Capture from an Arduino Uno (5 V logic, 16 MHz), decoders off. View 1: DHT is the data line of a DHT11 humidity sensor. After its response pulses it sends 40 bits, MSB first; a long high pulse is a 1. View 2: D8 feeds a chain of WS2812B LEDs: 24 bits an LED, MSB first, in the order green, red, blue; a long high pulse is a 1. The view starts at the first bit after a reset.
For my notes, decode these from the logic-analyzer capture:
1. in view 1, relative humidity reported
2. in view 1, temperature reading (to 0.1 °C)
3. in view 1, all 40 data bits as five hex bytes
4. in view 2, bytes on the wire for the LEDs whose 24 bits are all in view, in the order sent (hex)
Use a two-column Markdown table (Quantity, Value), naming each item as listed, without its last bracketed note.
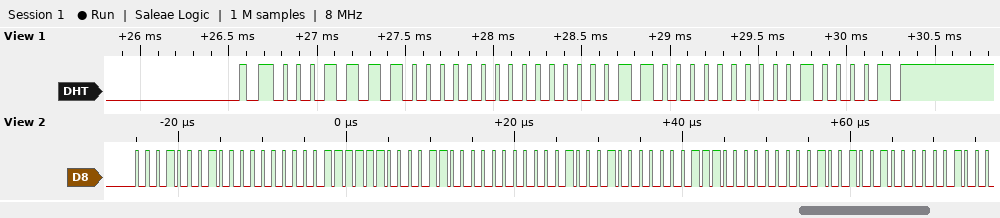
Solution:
| Quantity | Value |
|---|---|
| in view 1, relative humidity reported | 30 % |
| in view 1, temperature reading | 3.0 °C |
| in view 1, all 40 data bits as five hex bytes | 1E 00 03 00 21 |
| in view 2, bytes on the wire for the LEDs whose 24 bits are all in view, in the order sent | 11 00 3F 0C 00 44 07 00 49 |
